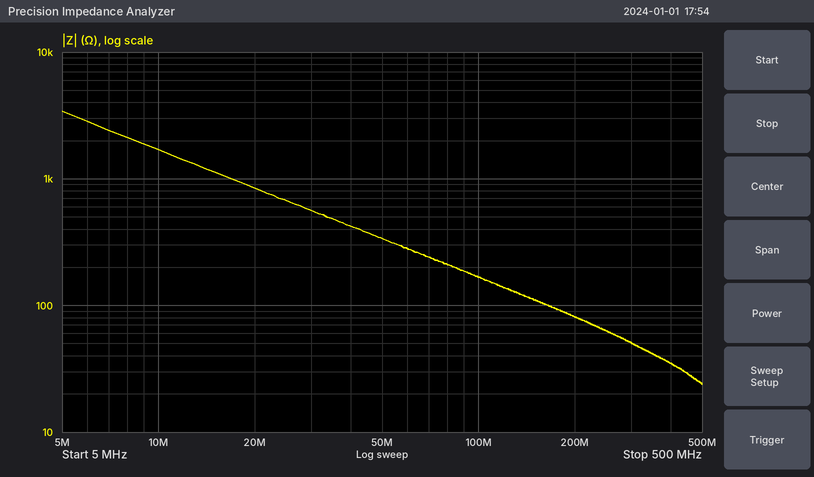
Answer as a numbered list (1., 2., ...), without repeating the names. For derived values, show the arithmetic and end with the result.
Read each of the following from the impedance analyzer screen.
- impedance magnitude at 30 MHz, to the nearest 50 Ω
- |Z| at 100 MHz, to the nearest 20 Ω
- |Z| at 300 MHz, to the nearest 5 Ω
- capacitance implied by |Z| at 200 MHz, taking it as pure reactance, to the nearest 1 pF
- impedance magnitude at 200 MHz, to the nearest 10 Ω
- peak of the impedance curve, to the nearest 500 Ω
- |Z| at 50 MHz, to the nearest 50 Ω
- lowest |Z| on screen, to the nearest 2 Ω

1. 550 Ω
2. 160 Ω
3. 50 Ω
4. C = 1/(2π × 200 MHz × 80 Ω) ≈ 10 pF
5. 80 Ω
6. 3.5 kΩ
7. 350 Ω
8. 24 Ω
